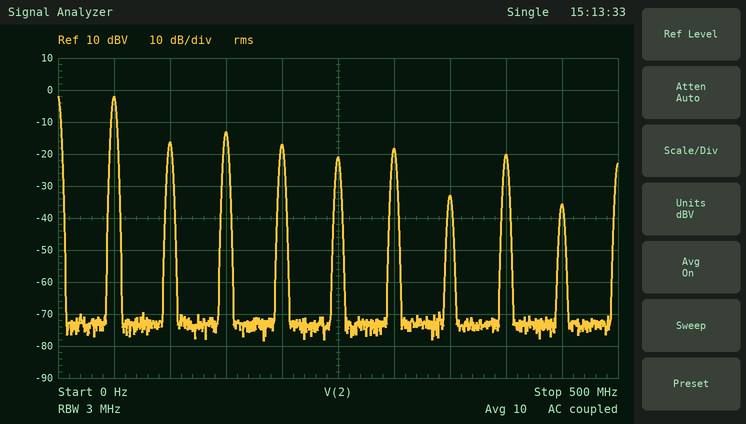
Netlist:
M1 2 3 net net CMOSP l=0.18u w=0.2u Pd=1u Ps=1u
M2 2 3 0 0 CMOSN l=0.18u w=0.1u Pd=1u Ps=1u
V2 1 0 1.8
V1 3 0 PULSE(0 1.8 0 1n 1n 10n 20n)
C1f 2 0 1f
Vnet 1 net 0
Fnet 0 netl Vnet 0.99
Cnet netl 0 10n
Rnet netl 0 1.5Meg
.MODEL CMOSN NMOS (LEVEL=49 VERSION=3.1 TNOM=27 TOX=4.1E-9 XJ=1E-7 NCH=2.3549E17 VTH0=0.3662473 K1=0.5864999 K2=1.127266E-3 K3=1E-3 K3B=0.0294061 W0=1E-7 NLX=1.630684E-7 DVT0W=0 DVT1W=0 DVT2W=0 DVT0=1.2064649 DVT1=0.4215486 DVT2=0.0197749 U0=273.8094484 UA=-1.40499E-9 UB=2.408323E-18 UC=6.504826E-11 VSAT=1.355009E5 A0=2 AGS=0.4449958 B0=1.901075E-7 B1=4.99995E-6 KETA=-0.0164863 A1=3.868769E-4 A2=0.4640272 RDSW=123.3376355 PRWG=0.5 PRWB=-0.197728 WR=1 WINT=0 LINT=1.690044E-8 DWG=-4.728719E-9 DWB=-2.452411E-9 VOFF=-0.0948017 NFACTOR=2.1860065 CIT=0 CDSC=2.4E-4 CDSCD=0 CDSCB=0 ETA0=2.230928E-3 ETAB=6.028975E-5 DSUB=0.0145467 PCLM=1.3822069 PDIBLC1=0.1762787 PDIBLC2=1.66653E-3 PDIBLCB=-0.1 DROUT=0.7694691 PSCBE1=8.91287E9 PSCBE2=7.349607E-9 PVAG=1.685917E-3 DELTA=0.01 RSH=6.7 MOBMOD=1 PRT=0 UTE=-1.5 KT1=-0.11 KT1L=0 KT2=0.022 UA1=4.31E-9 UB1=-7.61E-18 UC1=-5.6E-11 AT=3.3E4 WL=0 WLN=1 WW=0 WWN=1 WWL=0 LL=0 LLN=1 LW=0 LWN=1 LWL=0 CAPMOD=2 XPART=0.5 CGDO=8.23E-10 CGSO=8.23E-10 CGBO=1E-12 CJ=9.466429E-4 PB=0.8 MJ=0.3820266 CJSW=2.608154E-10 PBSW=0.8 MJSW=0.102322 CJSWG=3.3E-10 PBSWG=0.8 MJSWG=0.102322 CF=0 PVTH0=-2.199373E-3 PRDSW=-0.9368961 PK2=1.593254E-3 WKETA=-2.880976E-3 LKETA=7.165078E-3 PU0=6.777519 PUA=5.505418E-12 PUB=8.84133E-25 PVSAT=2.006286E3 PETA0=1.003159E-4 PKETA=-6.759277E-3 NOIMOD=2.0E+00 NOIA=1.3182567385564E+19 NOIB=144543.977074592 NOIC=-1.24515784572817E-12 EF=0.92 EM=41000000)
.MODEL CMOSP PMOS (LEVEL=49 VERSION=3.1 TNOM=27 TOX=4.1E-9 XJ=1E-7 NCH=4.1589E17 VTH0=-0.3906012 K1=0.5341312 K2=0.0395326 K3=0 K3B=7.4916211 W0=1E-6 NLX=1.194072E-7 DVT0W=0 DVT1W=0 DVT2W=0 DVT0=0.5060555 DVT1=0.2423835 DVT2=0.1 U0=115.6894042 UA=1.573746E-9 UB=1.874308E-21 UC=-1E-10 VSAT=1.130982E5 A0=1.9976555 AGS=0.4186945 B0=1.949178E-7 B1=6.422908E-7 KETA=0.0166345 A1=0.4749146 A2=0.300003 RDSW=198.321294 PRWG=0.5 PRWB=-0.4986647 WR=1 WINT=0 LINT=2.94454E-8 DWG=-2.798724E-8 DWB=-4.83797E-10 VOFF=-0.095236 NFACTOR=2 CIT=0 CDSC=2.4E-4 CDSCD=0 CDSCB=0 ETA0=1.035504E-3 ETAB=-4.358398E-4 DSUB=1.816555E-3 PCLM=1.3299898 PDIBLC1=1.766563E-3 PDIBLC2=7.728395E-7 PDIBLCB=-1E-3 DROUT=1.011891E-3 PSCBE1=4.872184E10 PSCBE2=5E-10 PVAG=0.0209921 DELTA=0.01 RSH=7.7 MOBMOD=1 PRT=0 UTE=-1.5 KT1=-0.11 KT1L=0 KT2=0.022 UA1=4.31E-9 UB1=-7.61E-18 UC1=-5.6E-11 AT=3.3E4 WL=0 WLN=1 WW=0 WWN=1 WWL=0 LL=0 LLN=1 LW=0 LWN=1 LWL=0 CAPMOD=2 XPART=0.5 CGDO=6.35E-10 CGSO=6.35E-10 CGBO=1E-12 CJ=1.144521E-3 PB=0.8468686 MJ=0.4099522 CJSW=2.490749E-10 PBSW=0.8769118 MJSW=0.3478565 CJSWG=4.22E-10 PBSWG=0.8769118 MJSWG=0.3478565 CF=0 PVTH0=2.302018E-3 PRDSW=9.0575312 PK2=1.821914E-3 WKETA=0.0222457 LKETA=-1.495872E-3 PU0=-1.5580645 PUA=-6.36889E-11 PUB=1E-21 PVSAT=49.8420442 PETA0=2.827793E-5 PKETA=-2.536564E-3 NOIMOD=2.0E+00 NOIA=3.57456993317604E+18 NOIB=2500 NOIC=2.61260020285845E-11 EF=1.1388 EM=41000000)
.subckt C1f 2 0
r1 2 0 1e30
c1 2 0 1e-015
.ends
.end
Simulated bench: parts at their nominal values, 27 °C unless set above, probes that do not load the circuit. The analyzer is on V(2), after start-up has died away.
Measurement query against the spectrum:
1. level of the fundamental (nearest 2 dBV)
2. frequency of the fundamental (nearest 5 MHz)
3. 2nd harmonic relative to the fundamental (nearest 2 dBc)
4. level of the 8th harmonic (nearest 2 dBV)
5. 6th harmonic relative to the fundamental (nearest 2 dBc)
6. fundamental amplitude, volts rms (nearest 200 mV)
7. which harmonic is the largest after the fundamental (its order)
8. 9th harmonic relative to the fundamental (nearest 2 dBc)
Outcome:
-2 dBV
50 MHz
-14 dBc
-20 dBV
-16 dBc
800 mV
3
-34 dBc
